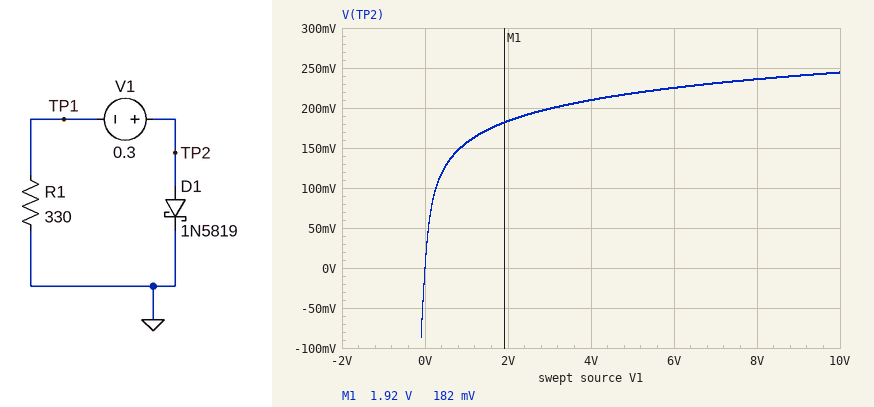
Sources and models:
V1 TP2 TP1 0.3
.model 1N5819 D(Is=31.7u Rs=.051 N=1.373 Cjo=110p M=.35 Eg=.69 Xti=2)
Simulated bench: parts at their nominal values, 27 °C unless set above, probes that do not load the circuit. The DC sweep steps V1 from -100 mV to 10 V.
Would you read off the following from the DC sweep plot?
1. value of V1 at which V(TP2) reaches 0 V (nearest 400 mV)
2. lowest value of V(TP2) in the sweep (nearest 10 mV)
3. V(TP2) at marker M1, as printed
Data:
0 V
-90 mV
182 mV
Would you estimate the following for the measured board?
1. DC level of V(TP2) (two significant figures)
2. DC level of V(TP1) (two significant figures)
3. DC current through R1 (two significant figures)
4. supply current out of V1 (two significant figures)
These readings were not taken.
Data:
110 mV
-190 mV
590 µA
590 µA
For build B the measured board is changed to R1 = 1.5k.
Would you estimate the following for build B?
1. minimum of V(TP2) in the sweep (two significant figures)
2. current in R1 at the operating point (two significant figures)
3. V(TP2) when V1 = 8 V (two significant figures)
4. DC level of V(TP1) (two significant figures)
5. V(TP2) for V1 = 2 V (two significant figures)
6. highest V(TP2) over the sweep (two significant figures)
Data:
-61 mV
160 µA
180 mV
-240 mV
130 mV
190 mV
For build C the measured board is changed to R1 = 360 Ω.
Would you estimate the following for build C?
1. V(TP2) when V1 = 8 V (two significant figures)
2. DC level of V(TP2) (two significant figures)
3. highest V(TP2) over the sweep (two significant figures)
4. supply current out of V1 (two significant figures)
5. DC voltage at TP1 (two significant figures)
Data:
230 mV
100 mV
240 mV
550 µA
-200 mV
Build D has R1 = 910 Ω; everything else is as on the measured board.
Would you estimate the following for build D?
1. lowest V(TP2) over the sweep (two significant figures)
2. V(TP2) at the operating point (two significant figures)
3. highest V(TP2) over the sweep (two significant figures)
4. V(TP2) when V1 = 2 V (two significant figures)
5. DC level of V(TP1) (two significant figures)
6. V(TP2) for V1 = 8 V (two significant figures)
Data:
-75 mV
77 mV
210 mV
150 mV
-220 mV
200 mV
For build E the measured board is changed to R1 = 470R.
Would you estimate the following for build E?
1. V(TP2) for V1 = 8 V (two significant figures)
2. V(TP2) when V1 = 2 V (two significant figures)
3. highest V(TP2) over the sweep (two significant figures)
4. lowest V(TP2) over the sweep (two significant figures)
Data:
220 mV
170 mV
230 mV
-86 mV
